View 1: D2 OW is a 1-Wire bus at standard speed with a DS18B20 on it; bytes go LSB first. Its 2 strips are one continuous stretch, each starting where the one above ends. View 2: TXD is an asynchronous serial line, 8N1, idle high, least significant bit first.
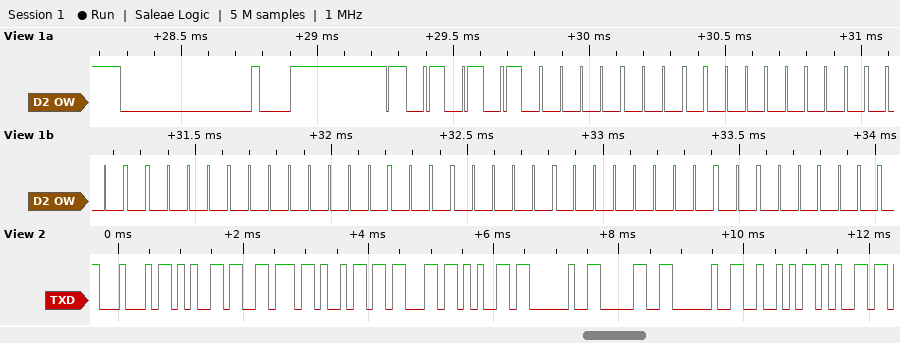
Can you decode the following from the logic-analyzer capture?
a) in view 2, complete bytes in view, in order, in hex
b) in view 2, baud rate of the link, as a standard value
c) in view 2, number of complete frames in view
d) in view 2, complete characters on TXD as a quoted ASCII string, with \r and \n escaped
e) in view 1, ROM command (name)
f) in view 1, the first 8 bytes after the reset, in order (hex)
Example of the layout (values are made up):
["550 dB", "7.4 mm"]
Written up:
["44 65 76 69 63 65 20 30 20 52 65", "9600 baud", "11", "\"Device 0 Re\"", "Match ROM", "55 00 00 00 00 00 00 00"]
